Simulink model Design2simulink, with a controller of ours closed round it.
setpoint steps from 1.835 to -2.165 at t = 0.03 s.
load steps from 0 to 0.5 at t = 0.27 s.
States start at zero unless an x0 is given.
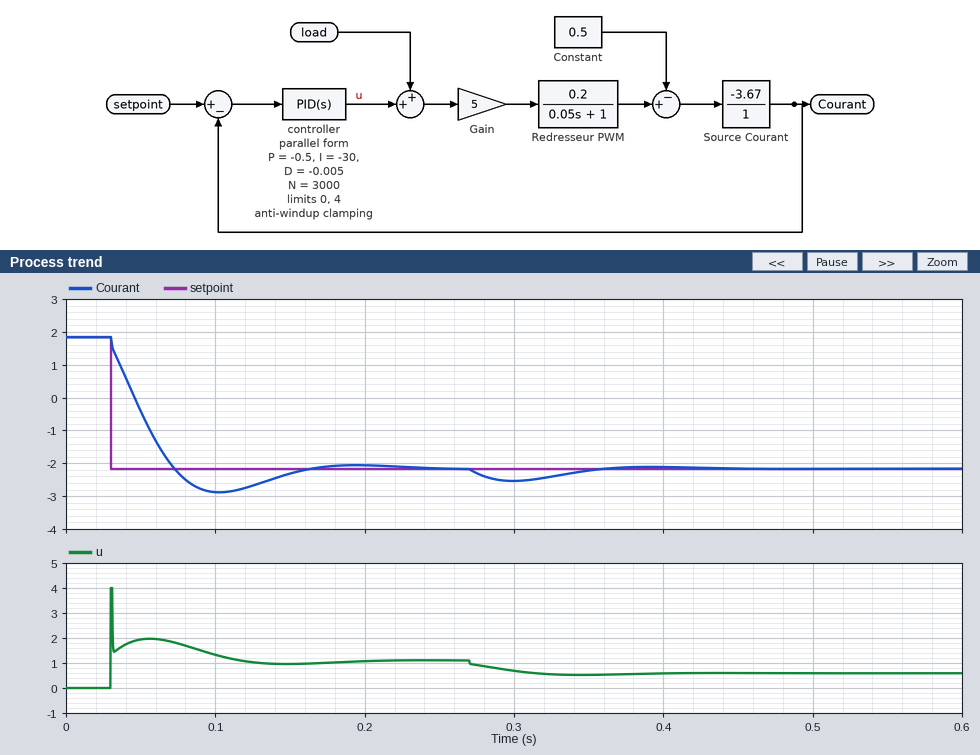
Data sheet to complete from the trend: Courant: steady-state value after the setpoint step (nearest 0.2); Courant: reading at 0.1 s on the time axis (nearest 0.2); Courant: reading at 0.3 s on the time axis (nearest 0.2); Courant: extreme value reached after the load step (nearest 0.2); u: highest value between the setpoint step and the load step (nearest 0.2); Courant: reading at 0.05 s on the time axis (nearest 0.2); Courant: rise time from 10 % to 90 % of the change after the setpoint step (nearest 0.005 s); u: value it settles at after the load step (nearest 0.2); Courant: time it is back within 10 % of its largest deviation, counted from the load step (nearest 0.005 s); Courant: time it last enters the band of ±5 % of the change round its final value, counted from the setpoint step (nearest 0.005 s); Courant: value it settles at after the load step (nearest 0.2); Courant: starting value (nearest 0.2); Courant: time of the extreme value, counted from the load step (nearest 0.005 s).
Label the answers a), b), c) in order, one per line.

a) -2.2
b) -2.8
c) -2.6
d) -2.6
e) 4.0
f) -0.4
g) 0.035 s
h) 0.6
i) 0.145 s
j) 0.115 s
k) -2.2
l) 1.8
m) 0.030 s
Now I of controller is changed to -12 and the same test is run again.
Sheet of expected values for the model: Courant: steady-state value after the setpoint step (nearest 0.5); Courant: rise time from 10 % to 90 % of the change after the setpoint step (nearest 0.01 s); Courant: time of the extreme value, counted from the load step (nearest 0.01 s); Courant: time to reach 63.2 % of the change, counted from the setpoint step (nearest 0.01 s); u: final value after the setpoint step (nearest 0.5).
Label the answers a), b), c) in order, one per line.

a) -2.0
b) 0.06 s
c) 0.04 s
d) 0.03 s
e) 1.0
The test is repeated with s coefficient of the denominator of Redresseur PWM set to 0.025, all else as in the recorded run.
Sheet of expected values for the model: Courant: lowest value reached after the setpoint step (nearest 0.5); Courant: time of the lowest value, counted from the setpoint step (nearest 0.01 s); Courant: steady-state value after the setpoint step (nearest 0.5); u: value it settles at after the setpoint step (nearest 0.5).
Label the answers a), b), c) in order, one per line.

a) -2.5
b) 0.06 s
c) -2.0
d) 1.0
